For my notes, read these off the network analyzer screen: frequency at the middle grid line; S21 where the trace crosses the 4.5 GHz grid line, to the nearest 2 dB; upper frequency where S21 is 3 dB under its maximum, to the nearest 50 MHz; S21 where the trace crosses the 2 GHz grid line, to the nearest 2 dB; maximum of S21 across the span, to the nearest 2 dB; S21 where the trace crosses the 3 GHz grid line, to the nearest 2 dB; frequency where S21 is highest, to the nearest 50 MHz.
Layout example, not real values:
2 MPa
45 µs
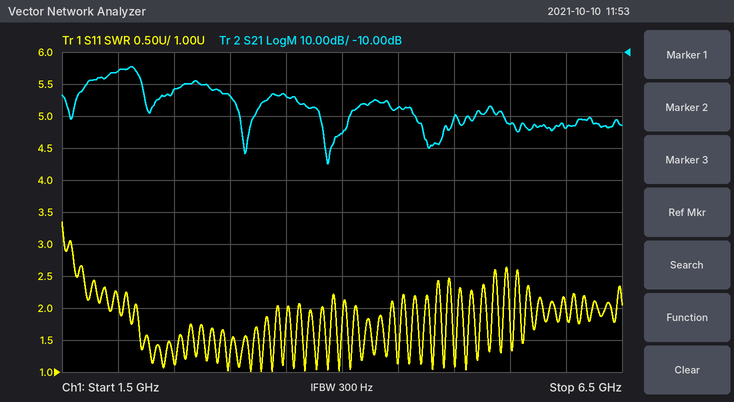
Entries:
4 GHz
-28 dB
2.20 GHz
-16 dB
-14 dB
-24 dB
2.10 GHz
